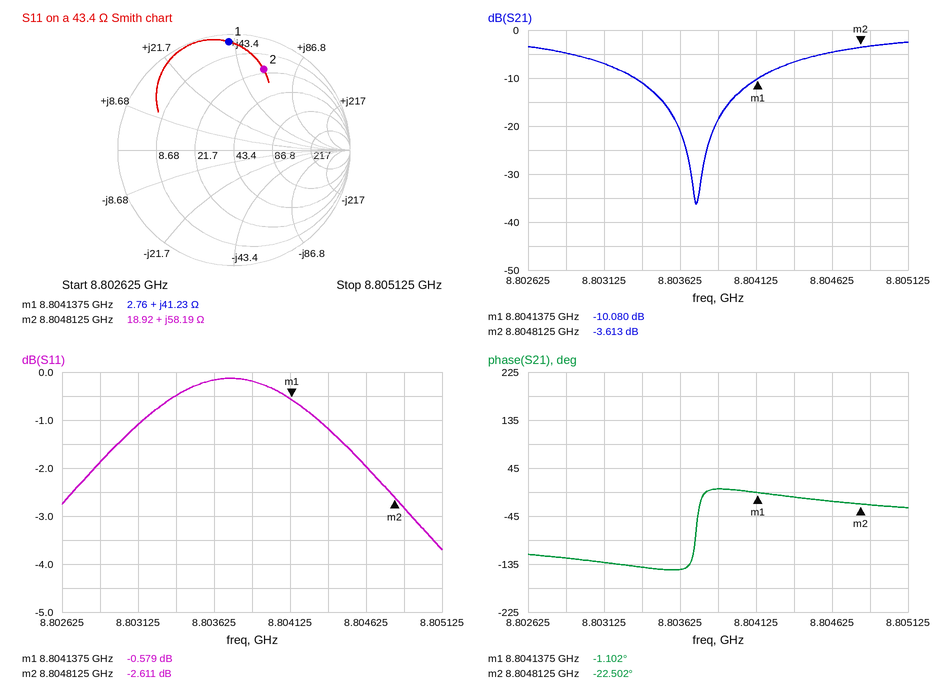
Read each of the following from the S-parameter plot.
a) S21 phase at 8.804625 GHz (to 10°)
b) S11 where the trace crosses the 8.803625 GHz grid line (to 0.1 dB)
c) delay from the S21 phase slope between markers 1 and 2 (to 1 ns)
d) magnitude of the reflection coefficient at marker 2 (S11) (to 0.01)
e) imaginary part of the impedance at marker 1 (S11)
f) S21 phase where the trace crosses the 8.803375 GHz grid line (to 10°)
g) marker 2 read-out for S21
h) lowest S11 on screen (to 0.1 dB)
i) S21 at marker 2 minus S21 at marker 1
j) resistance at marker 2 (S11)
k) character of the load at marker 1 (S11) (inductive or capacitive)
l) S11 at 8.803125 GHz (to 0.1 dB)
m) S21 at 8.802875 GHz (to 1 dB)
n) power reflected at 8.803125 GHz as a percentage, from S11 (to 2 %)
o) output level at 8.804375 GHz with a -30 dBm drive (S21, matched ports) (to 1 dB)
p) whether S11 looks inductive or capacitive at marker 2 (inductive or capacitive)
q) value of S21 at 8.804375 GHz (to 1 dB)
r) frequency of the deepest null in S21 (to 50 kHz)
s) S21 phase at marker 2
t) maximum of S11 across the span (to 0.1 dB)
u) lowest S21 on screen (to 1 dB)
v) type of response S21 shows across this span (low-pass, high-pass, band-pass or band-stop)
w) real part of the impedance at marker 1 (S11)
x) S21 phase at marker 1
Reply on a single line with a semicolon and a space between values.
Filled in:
-20°; -0.2 dB; 88 ns; 0.74; +41.23 Ω; -140°; -3.613 dB; -3.7 dB; 6.467 dB; 18.92 Ω; inductive; -1.1 dB; -5 dB; 78 %; -37 dBm; inductive; -7 dB; 8.80375 GHz; -22.502°; -0.1 dB; -36 dB; band-stop; 2.76 Ω; -1.102°
